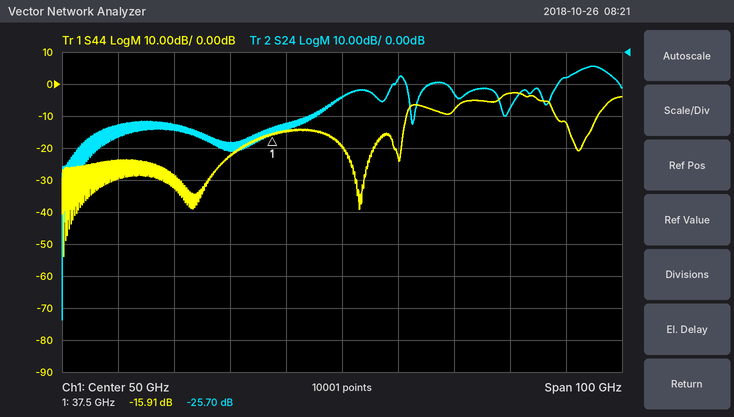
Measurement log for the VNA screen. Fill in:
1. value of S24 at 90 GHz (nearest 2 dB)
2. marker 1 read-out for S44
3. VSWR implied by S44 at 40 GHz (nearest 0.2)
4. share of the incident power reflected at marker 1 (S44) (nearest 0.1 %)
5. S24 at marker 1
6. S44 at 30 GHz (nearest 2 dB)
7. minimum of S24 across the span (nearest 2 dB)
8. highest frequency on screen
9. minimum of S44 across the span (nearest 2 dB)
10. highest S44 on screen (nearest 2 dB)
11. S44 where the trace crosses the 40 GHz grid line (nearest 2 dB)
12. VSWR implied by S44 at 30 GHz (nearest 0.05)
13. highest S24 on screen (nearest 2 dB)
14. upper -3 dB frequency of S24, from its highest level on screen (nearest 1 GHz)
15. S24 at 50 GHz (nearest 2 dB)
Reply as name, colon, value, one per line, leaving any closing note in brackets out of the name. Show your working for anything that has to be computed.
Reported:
value of S24 at 90 GHz: -8 dB
marker 1 read-out for S44: -15.91 dB
VSWR implied by S44 at 40 GHz: |Γ| = 10^(-14/20) = 0.1995; VSWR = (1 + 0.1995)/(1 − 0.1995) ≈ 1.50, so 1.4 to the nearest 0.2
share of the incident power reflected at marker 1 (S44): 10^(-15.91/10) ≈ 2.6 %
S24 at marker 1: -25.70 dB
S44 at 30 GHz: -22 dB
minimum of S24 across the span: -84 dB
highest frequency on screen: 100 GHz
minimum of S44 across the span: -54 dB
highest S44 on screen: -2 dB
S44 where the trace crosses the 40 GHz grid line: -14 dB
VSWR implied by S44 at 30 GHz: |Γ| = 10^(-22/20) = 0.0794; VSWR = (1 + 0.0794)/(1 − 0.0794) ≈ 1.17, so 1.15 to the nearest 0.05
highest S24 on screen: -4 dB
upper -3 dB frequency of S24, from its highest level on screen: 98 GHz
S24 at 50 GHz: -14 dB
